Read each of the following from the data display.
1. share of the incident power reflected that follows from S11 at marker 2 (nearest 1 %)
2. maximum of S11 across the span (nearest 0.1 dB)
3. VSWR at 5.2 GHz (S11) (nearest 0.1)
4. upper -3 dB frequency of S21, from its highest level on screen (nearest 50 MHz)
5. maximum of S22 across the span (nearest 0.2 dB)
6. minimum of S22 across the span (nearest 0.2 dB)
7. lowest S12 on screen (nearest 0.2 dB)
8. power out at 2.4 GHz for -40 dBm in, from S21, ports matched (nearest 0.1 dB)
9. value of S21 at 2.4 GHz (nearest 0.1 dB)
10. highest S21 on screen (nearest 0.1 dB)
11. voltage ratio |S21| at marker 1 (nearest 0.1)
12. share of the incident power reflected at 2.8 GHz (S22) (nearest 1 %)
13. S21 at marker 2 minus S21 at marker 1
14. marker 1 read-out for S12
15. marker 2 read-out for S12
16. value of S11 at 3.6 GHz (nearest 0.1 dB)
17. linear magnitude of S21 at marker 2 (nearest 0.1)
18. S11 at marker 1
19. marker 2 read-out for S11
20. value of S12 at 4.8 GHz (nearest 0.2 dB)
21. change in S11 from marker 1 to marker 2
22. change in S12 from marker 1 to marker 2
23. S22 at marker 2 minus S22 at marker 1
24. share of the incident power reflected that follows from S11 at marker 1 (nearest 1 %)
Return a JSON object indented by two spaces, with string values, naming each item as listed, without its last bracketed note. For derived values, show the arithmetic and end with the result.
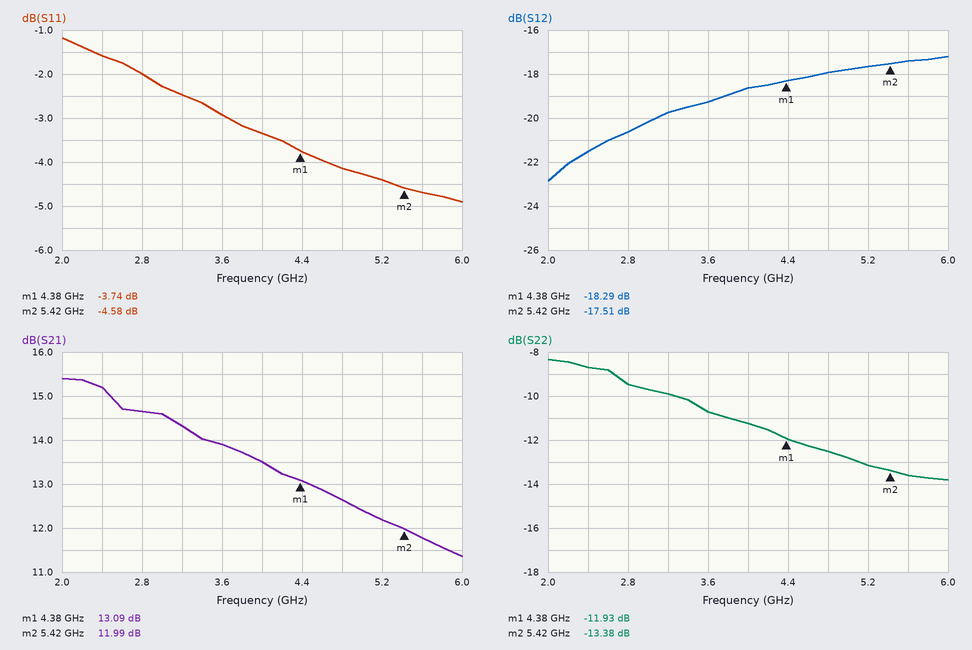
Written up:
{
  "share of the incident power reflected that follows from S11 at marker 2": "10^(-4.58/10) ≈ 35 %",
  "maximum of S11 across the span": "-1.2 dB",
  "VSWR at 5.2 GHz (S11)": "|Γ| = 10^(-4.4/20) = 0.6026; VSWR = (1 + 0.6026)/(1 − 0.6026) ≈ 4.0",
  "upper -3 dB frequency of S21, from its highest level on screen": "5.00 GHz",
  "maximum of S22 across the span": "-8.4 dB",
  "minimum of S22 across the span": "-13.8 dB",
  "lowest S12 on screen": "-22.8 dB",
  "power out at 2.4 GHz for -40 dBm in, from S21, ports matched": "-40 dBm + (15.2 dB) = -24.8 dBm",
  "value of S21 at 2.4 GHz": "15.2 dB",
  "highest S21 on screen": "15.4 dB",
  "voltage ratio |S21| at marker 1": "10^(13.09/20) ≈ 4.5",
  "share of the incident power reflected at 2.8 GHz (S22)": "10^(-9.4/10) ≈ 11 %",
  "S21 at marker 2 minus S21 at marker 1": "11.99 − (13.09) = -1.10 dB",
  "marker 1 read-out for S12": "-18.29 dB",
  "marker 2 read-out for S12": "-17.51 dB",
  "value of S11 at 3.6 GHz": "-2.9 dB",
  "linear magnitude of S21 at marker 2": "10^(11.99/20) ≈ 4.0",
  "S11 at marker 1": "-3.74 dB",
  "marker 2 read-out for S11": "-4.58 dB",
  "value of S12 at 4.8 GHz": "-18.0 dB",
  "change in S11 from marker 1 to marker 2": "-4.58 − (-3.74) = -0.84 dB",
  "change in S12 from marker 1 to marker 2": "-17.51 − (-18.29) = 0.78 dB",
  "S22 at marker 2 minus S22 at marker 1": "-13.38 − (-11.93) = -1.45 dB",
  "share of the incident power reflected that follows from S11 at marker 1": "10^(-3.74/10) ≈ 42 %"
}
